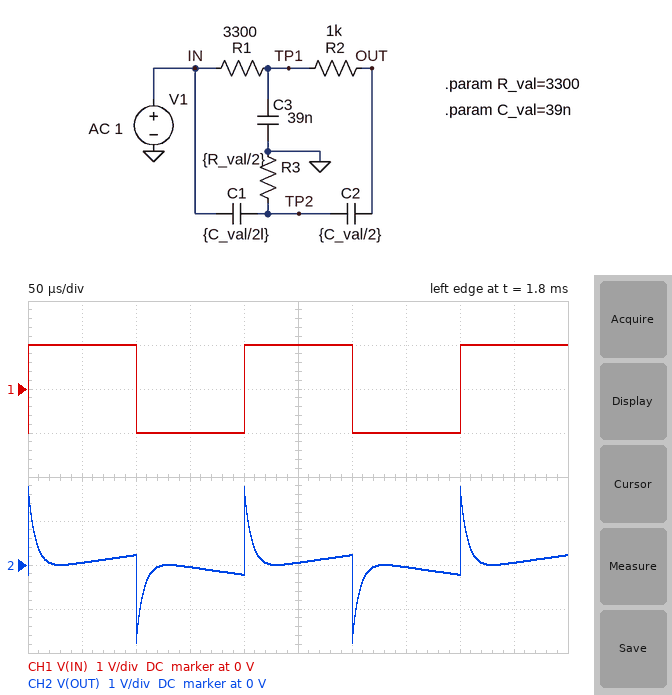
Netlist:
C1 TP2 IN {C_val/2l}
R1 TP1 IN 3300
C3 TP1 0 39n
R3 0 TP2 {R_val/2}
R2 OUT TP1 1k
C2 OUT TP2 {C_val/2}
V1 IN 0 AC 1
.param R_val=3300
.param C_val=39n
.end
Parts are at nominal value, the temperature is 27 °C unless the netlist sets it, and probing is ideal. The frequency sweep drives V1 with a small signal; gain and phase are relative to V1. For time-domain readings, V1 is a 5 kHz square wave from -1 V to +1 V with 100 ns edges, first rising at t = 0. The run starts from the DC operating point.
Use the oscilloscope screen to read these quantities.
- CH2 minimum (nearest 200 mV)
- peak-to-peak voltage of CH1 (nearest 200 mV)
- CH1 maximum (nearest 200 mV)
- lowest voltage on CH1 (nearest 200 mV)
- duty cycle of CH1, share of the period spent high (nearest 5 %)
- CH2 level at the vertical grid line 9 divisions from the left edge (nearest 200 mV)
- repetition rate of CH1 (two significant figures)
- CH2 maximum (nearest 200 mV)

-1.8 V
2.0 V
1.0 V
-1.0 V
50 %
0 V
5.0 kHz
1.8 V
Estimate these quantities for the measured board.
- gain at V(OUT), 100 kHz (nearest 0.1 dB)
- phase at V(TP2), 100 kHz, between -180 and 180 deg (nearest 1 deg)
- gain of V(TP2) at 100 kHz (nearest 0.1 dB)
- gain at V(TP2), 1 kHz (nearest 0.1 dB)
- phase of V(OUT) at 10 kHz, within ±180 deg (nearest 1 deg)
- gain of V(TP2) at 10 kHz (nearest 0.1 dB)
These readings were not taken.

-0.2 dB
7 deg
-0.2 dB
-11.6 dB
56 deg
-4.4 dB
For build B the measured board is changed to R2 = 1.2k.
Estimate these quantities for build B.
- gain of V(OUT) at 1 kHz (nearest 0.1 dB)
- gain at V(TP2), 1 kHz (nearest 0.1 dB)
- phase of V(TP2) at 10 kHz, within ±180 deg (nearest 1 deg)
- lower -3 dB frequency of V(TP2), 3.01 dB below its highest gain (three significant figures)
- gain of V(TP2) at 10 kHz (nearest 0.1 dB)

-5.4 dB
-11.7 dB
29 deg
14.5 kHz
-4.2 dB
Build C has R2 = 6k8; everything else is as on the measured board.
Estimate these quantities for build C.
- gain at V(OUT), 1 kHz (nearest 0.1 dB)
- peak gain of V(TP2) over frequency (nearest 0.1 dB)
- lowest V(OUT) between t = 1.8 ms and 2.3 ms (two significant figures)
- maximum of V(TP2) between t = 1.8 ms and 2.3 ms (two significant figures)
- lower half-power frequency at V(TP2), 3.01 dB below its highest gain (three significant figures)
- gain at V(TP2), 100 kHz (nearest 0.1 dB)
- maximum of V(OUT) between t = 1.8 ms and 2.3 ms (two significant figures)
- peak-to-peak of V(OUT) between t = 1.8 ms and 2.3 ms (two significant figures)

-9.3 dB
0 dB
-2.0 V
1.9 V
6.75 kHz
0 dB
2.0 V
3.9 V
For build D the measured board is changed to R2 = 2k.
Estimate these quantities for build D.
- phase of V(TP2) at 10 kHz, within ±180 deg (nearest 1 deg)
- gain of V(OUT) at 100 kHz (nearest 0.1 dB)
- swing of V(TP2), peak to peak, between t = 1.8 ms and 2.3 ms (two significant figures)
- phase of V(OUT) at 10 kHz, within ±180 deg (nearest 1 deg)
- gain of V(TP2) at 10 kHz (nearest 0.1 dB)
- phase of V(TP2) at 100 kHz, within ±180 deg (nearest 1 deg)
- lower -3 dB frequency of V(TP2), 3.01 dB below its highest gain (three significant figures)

32 deg
-0.1 dB
3.6 V
53 deg
-3.3 dB
5 deg
10.8 kHz
